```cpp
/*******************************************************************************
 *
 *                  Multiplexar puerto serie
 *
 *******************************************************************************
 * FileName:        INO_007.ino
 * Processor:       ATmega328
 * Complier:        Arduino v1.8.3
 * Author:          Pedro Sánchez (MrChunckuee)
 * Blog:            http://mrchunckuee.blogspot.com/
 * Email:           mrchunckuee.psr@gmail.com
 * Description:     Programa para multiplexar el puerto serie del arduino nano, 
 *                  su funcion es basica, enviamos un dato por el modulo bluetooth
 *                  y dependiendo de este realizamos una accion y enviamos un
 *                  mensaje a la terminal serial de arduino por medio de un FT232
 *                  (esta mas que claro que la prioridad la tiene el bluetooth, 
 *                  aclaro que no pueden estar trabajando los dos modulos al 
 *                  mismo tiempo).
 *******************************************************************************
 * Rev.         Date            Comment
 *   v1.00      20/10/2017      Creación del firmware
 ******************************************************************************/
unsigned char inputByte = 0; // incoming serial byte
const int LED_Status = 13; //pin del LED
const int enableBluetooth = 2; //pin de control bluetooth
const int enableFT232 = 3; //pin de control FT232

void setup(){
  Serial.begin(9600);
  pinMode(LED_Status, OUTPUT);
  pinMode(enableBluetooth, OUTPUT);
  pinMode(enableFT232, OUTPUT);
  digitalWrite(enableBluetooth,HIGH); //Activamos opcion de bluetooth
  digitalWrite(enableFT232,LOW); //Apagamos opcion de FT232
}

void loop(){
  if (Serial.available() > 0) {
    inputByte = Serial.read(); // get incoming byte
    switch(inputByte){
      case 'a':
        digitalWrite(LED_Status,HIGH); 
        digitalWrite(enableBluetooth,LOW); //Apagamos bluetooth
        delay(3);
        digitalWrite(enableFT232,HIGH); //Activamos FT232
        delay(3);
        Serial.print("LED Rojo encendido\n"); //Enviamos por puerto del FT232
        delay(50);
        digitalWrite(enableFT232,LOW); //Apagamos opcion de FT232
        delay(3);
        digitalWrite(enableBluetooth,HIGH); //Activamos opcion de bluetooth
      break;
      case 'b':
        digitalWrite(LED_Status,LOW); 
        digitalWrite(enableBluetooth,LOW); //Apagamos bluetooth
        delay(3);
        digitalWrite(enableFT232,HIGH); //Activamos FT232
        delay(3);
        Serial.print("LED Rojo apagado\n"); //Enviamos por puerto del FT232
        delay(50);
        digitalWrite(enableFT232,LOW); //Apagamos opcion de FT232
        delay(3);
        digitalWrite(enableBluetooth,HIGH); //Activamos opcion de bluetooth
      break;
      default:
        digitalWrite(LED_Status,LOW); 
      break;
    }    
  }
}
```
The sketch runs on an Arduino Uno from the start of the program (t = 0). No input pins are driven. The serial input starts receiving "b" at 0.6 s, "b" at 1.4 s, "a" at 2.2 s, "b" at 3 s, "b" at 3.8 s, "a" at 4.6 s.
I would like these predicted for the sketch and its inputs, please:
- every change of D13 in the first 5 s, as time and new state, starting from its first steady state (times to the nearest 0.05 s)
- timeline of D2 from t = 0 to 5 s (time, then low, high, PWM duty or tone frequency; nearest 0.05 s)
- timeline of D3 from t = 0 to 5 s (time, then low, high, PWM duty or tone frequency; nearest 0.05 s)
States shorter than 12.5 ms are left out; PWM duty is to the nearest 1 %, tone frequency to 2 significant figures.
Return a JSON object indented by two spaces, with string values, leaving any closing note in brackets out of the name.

{
  "every change of D13 in the first 5 s, as time and new state, starting from its first steady state": "0 s low; 2.2 s high; 3 s low; 4.6 s high",
  "timeline of D2 from t = 0 to 5 s": "0 s high; 0.6 s low; 0.65 s high; 1.4 s low; 1.45 s high; 2.2 s low; 2.25 s high; 3 s low; 3.05 s high; 3.8 s low; 3.85 s high; 4.6 s low; 4.65 s high",
  "timeline of D3 from t = 0 to 5 s": "0 s low; 0.6 s high; 0.65 s low; 1.4 s high; 1.45 s low; 2.2 s high; 2.25 s low; 3 s high; 3.05 s low; 3.8 s high; 3.85 s low; 4.6 s high; 4.65 s low"
}
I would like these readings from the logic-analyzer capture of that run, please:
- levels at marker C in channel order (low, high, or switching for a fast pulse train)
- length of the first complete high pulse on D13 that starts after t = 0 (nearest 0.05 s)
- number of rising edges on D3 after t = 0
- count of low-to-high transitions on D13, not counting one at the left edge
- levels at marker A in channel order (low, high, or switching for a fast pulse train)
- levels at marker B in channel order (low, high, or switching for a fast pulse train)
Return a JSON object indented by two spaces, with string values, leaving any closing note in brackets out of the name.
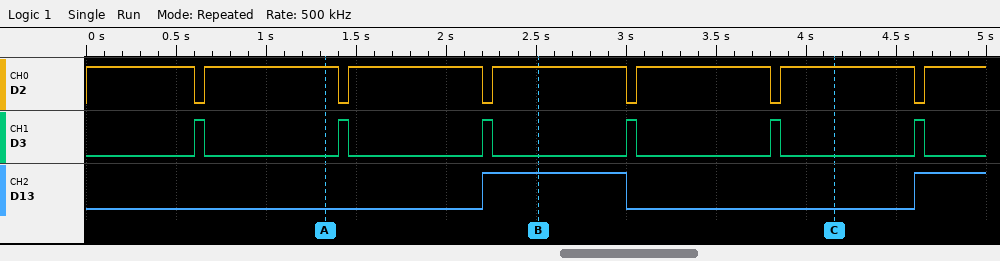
{
  "levels at marker C in channel order": "D2 high, D3 low, D13 low",
  "length of the first complete high pulse on D13 that starts after t = 0": "0.80 s",
  "number of rising edges on D3 after t = 0": "6",
  "count of low-to-high transitions on D13, not counting one at the left edge": "2",
  "levels at marker A in channel order": "D2 high, D3 low, D13 low",
  "levels at marker B in channel order": "D2 high, D3 low, D13 high"
}
